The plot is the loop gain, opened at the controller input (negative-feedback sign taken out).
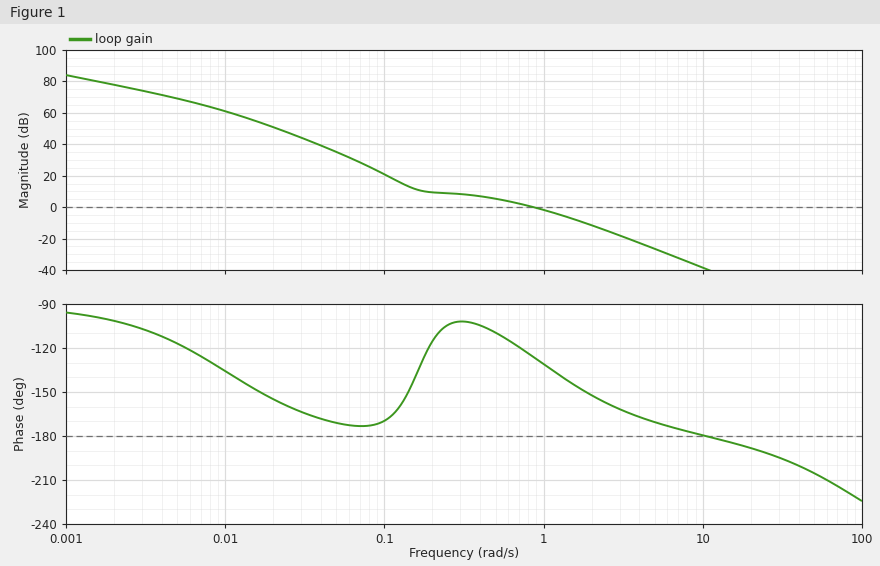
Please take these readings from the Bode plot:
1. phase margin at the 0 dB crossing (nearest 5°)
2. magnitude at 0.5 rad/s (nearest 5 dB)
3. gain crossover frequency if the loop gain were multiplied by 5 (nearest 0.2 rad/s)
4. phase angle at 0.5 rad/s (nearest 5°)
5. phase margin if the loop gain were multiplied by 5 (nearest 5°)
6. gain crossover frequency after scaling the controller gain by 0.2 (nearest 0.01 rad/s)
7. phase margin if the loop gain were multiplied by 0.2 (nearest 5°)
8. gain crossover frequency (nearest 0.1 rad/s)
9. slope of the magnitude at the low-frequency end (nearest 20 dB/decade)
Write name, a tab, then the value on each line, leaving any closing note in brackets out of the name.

phase margin at the 0 dB crossing	55°
magnitude at 0.5 rad/s	5 dB
gain crossover frequency if the loop gain were multiplied by 5	2.4 rad/s
phase angle at 0.5 rad/s	-110°
phase margin if the loop gain were multiplied by 5	25°
gain crossover frequency after scaling the controller gain by 0.2	0.14 rad/s
phase margin if the loop gain were multiplied by 0.2	25°
gain crossover frequency	0.9 rad/s
slope of the magnitude at the low-frequency end	-20 dB/decade
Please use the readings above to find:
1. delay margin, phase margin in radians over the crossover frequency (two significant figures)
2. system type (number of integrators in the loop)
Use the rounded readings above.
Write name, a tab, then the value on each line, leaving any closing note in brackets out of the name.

delay margin, phase margin in radians over the crossover frequency	1.1 s
system type	1
